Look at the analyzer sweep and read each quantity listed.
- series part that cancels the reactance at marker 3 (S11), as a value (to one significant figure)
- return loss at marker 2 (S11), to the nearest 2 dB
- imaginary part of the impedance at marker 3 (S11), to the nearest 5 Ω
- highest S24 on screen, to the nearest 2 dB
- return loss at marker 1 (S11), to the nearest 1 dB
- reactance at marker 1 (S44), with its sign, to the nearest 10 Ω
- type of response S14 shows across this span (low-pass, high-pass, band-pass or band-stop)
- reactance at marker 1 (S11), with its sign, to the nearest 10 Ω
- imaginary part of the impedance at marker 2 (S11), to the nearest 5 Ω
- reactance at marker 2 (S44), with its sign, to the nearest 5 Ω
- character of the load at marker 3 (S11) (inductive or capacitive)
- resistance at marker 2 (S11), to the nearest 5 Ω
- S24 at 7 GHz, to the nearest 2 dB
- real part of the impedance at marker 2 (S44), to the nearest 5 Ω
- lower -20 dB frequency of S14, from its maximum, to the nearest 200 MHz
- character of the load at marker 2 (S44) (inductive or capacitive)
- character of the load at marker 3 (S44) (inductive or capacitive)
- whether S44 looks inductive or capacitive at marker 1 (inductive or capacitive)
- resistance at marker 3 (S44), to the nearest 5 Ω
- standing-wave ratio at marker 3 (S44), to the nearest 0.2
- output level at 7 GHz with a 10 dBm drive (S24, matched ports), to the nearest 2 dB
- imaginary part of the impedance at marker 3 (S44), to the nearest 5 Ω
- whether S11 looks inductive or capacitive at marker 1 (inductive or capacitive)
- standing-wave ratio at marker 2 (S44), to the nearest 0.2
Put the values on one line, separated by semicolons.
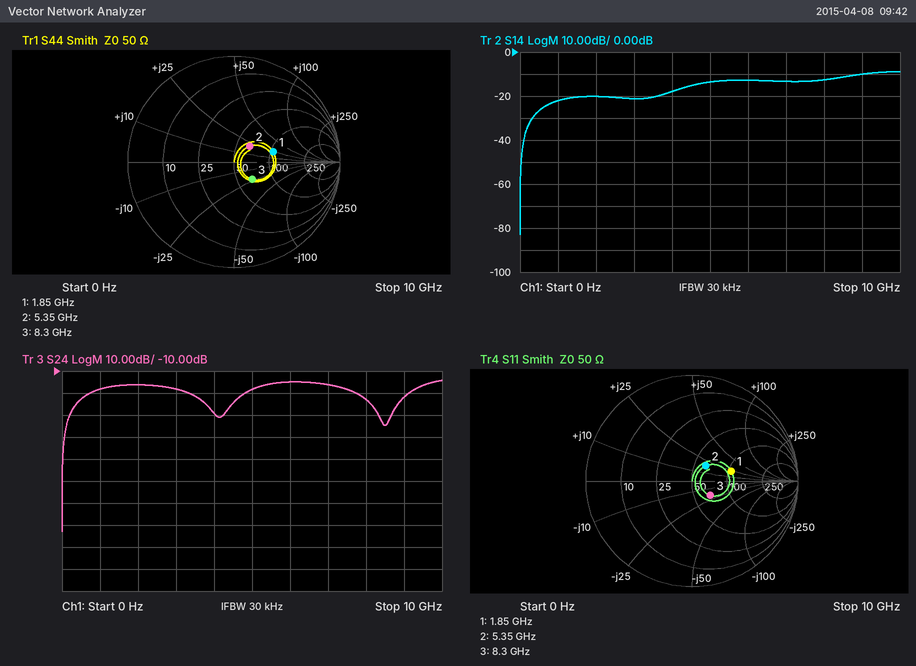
400 pH; 14 dB; -20 Ω; -14 dB; 8 dB; +20 Ω; high-pass; +20 Ω; +20 Ω; +20 Ω; capacitive; 60 Ω; -16 dB; 65 Ω; 400 MHz; inductive; capacitive; inductive; 65 Ω; 1.6; -6 dBm; -25 Ω; inductive; 1.6
